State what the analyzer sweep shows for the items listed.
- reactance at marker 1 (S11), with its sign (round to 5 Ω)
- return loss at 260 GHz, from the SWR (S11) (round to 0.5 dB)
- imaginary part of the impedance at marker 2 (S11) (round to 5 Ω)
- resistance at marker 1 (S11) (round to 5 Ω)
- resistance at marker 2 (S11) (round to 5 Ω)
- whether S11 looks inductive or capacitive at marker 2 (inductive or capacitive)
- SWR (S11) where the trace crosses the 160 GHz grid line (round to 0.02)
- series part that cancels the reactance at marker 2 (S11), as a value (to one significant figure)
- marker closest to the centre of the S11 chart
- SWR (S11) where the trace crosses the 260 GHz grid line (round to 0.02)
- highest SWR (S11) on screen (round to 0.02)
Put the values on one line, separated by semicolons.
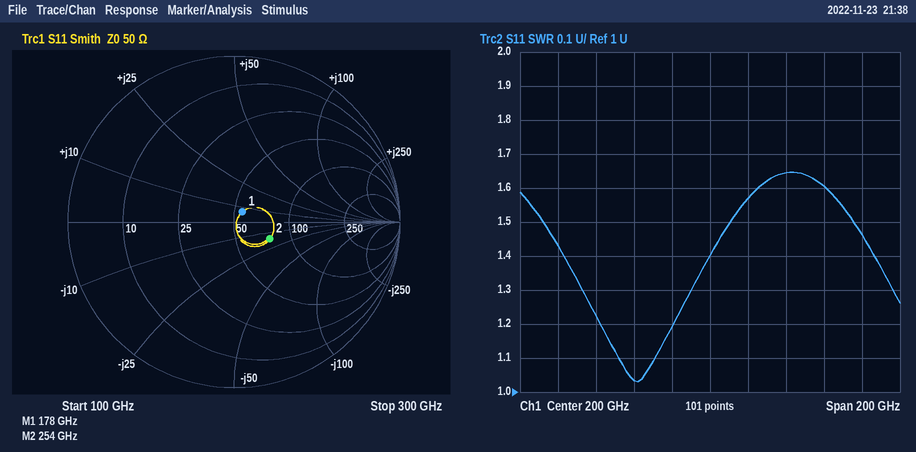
+5 Ω; 12.5 dB; -15 Ω; 55 Ω; 75 Ω; capacitive; 1.04; 10 pH; marker 1; 1.60; 1.64
